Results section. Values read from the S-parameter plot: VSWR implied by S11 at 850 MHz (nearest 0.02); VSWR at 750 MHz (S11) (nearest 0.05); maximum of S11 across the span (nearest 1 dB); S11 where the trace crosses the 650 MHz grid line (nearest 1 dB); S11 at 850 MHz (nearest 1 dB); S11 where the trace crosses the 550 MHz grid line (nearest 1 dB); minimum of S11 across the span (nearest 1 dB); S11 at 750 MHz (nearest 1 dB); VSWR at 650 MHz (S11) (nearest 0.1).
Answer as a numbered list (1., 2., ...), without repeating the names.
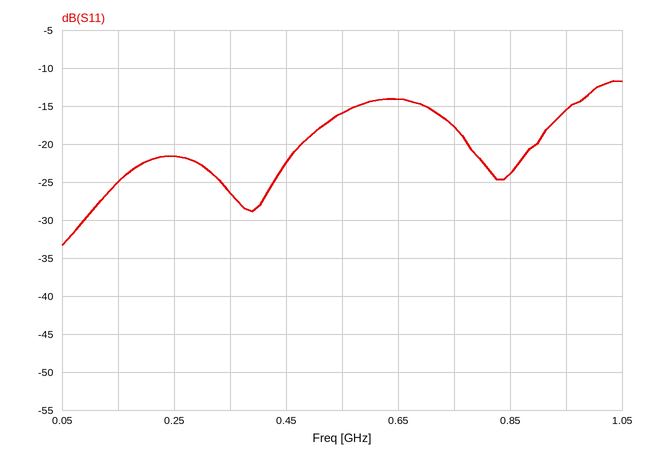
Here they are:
1. 1.14
2. 1.30
3. -12 dB
4. -14 dB
5. -24 dB
6. -16 dB
7. -33 dB
8. -18 dB
9. 1.5
